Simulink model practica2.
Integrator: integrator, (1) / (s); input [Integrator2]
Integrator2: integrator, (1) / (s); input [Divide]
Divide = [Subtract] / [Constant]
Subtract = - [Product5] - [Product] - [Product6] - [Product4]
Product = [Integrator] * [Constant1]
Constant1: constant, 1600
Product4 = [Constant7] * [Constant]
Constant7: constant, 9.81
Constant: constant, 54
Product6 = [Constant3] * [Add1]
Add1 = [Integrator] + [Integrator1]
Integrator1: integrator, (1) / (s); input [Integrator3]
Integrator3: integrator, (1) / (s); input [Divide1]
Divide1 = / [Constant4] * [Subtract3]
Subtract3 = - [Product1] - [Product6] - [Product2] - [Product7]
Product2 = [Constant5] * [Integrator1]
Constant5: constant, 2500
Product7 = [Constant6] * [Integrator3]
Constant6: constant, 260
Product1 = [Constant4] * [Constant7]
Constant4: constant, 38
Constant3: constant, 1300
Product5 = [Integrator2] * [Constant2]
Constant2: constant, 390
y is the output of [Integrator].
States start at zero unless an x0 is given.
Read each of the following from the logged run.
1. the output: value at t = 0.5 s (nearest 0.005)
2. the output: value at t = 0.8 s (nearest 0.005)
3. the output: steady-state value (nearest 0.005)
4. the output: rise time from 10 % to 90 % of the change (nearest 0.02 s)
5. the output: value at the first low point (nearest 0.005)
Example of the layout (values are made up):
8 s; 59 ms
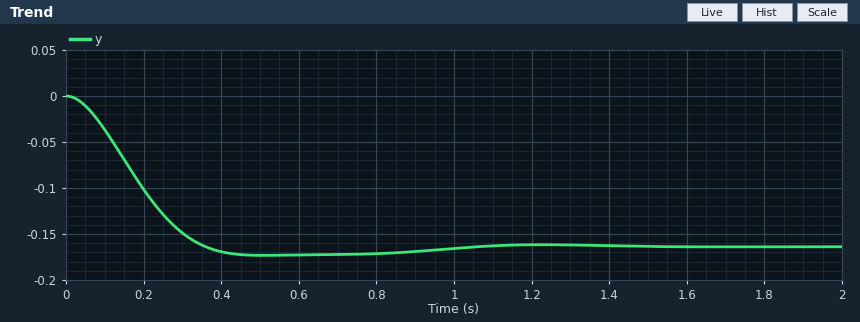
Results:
-0.175; -0.170; -0.165; 0.24 s; -0.175
